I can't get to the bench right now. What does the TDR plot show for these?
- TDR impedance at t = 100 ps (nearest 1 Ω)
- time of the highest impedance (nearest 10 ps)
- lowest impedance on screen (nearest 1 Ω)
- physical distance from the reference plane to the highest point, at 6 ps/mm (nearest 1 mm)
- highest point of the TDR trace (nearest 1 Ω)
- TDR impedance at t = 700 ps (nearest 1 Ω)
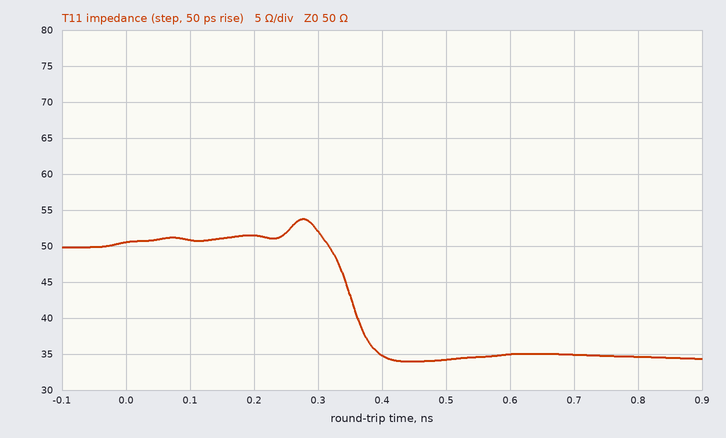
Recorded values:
51 Ω
280 ps
34 Ω
23 mm
54 Ω
35 Ω
